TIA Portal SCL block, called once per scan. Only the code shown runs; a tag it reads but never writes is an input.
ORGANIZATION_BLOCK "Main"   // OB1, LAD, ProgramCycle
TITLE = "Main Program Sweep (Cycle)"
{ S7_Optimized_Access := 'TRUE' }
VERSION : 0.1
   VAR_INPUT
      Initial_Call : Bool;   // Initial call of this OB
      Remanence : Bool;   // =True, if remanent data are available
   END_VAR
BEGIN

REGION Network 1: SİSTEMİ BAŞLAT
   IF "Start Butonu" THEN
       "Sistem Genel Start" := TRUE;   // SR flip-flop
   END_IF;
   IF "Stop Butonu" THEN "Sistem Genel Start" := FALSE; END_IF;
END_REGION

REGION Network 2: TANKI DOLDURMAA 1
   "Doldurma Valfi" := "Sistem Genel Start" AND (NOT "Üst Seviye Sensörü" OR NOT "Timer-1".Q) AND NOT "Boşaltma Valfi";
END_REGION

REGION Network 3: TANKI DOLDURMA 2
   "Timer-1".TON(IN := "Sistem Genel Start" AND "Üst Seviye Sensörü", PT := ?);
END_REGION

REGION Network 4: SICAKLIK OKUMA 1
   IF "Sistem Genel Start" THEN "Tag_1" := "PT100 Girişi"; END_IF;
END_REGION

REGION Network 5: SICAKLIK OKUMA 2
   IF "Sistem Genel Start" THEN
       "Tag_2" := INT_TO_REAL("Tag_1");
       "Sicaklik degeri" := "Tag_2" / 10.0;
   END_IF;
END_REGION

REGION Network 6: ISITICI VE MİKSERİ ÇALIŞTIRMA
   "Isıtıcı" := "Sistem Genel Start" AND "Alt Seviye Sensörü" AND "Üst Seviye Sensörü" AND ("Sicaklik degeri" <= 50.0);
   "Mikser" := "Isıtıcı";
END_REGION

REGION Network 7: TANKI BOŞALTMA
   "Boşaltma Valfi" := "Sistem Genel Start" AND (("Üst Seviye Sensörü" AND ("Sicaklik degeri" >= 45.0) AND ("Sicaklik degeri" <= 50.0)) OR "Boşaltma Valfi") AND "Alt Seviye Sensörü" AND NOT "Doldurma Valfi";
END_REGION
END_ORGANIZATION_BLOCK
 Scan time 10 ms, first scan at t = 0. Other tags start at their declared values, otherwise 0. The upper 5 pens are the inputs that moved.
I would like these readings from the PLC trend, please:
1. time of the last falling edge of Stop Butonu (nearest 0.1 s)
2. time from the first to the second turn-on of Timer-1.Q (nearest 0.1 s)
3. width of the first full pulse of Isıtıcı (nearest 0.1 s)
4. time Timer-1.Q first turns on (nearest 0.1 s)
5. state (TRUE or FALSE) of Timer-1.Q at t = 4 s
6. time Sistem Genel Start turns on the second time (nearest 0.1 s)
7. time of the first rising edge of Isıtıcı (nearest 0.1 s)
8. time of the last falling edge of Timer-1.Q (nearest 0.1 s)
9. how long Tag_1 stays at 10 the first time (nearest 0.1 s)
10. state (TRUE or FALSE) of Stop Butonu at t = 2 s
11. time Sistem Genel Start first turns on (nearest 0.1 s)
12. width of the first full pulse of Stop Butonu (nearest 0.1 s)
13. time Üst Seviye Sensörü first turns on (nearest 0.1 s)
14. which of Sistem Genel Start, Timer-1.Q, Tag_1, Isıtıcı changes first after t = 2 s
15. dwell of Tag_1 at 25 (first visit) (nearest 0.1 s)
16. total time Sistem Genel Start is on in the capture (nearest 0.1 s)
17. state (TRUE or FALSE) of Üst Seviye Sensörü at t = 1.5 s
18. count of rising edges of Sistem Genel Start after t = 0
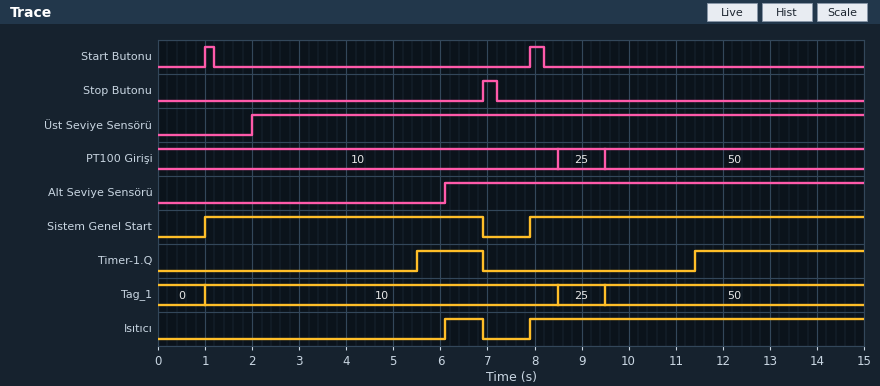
7.2 s
5.9 s
0.8 s
5.5 s
FALSE
7.9 s
6.1 s
6.9 s
7.5 s
FALSE
1.0 s
0.3 s
2.0 s
Timer-1.Q
1.0 s
13.0 s
FALSE
2
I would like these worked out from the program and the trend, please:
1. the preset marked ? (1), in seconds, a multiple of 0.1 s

3.5 s
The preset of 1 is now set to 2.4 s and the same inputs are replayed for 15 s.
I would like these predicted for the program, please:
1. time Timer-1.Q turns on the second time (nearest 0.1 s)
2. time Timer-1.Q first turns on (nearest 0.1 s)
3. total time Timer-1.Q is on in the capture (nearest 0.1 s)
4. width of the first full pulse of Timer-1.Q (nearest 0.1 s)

10.3 s
4.4 s
7.2 s
2.5 s
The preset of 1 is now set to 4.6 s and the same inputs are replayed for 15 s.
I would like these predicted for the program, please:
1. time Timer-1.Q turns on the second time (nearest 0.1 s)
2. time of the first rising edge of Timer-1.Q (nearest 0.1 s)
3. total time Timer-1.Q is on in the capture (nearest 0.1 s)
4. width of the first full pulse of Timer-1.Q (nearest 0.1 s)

12.5 s
6.6 s
2.8 s
0.3 s
